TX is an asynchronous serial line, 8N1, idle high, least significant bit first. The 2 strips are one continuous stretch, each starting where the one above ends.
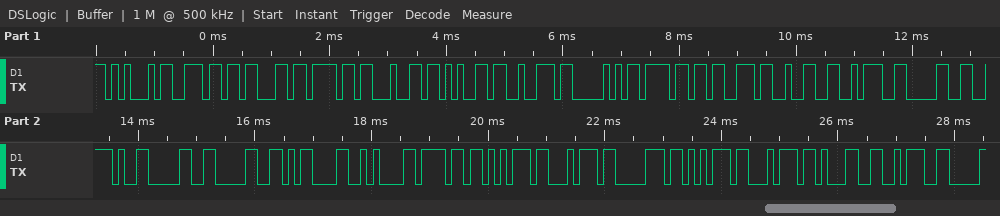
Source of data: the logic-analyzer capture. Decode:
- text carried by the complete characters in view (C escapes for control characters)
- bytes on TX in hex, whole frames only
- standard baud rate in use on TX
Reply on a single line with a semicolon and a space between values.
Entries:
"EncoderPos2:0.00\r\noutput1:"; 45 6E 63 6F 64 65 72 50 6F 73 32 3A 30 2E 30 30 0D 0A 6F 75 74 70 75 74 31 3A; 9600 baud
